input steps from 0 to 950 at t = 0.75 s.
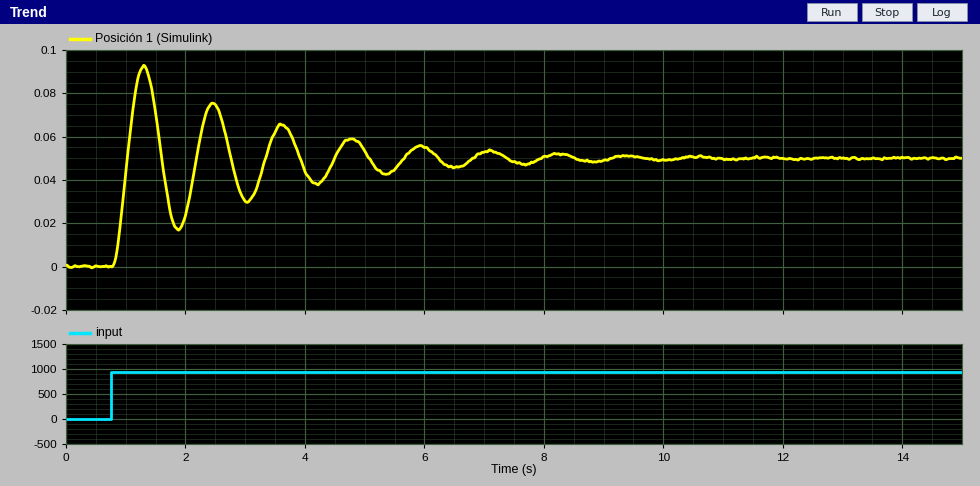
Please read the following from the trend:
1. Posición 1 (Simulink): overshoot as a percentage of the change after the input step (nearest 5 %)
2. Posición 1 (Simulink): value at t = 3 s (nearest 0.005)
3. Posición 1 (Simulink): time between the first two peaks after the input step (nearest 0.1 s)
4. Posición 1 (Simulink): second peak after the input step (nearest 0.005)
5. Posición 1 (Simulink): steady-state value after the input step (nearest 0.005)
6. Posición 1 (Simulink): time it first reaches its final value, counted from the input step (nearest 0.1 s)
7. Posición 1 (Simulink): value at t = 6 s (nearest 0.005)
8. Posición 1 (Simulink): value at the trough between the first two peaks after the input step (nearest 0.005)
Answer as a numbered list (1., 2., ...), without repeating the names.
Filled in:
1. 85 %
2. 0.030
3. 1.2 s
4. 0.075
5. 0.050
6. 0.3 s
7. 0.055
8. 0.015
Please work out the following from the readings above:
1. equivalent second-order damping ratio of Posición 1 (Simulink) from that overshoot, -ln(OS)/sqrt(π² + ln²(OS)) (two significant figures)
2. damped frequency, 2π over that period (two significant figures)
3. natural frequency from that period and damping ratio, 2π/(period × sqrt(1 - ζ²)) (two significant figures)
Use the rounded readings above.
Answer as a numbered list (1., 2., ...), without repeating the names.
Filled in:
1. 0.052
2. 5.2 rad/s
3. 5.2 rad/s
